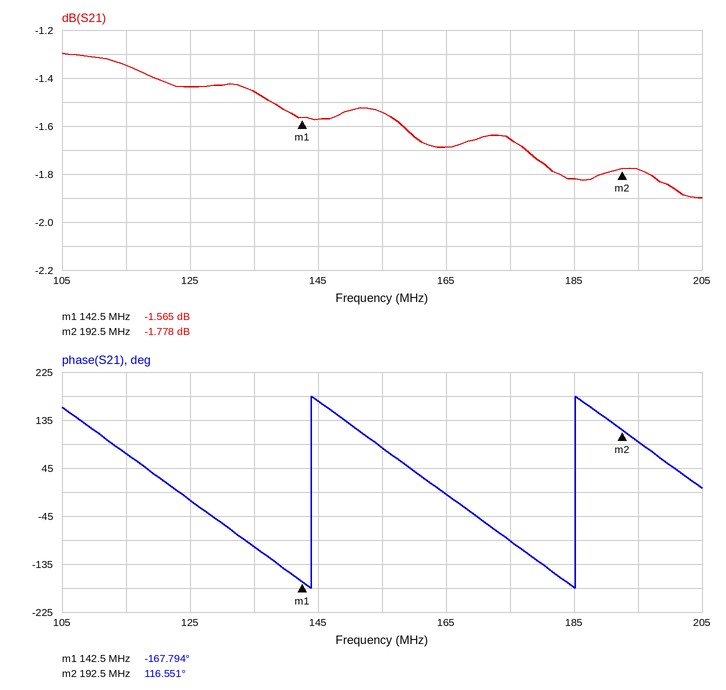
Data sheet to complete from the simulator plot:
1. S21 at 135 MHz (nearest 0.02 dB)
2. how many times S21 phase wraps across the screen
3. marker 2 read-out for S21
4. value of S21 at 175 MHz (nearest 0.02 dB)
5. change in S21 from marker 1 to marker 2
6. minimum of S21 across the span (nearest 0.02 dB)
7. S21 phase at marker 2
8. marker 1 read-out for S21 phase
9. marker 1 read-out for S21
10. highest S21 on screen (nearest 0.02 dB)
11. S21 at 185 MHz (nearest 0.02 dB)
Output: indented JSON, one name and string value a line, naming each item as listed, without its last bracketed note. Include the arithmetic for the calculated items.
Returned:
{
  "S21 at 135 MHz": "-1.46 dB",
  "how many times S21 phase wraps across the screen": "2",
  "marker 2 read-out for S21": "-1.778 dB",
  "value of S21 at 175 MHz": "-1.66 dB",
  "change in S21 from marker 1 to marker 2": "-1.778 − (-1.565) = -0.213 dB",
  "minimum of S21 across the span": "-1.90 dB",
  "S21 phase at marker 2": "116.551°",
  "marker 1 read-out for S21 phase": "-167.794°",
  "marker 1 read-out for S21": "-1.565 dB",
  "highest S21 on screen": "-1.30 dB",
  "S21 at 185 MHz": "-1.82 dB"
}
